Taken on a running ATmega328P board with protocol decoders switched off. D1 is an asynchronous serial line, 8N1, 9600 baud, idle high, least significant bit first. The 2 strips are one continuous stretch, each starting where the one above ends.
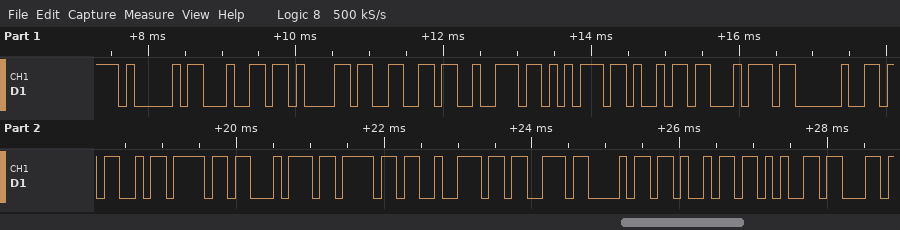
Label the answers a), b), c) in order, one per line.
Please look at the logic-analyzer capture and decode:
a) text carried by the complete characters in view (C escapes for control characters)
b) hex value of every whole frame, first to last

a) "Adafruit Motorshie"
b) 0x41 0x64 0x61 0x66 0x72 0x75 0x69 0x74 0x20 0x4D 0x6F 0x74 0x6F 0x72 0x73 0x68 0x69 0x65
